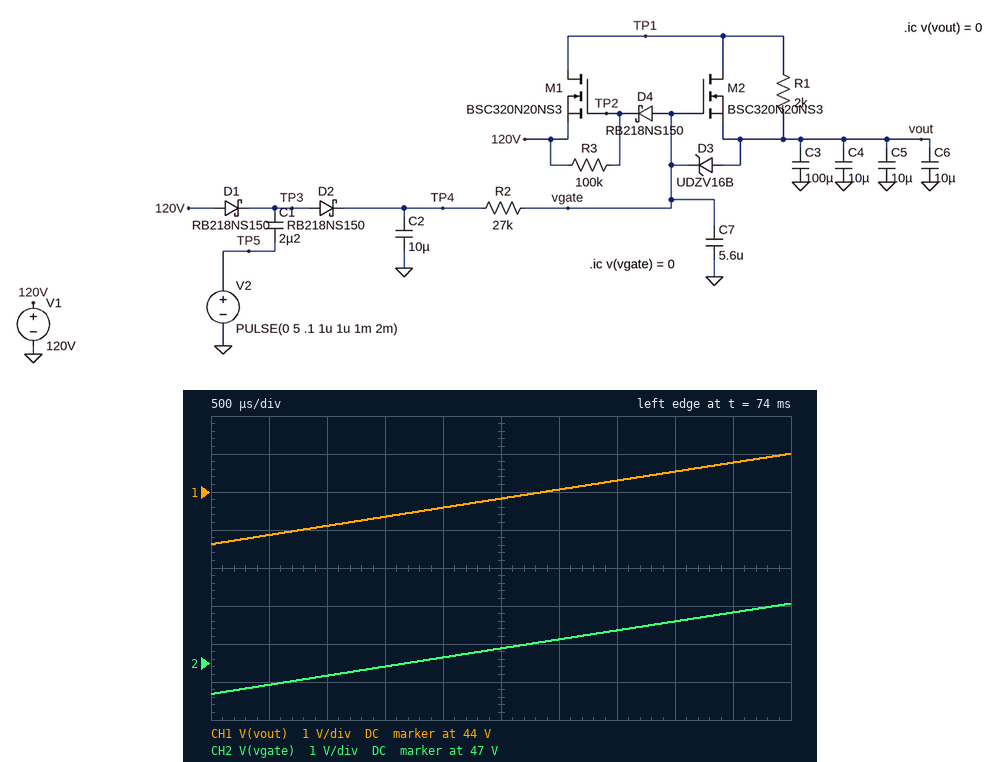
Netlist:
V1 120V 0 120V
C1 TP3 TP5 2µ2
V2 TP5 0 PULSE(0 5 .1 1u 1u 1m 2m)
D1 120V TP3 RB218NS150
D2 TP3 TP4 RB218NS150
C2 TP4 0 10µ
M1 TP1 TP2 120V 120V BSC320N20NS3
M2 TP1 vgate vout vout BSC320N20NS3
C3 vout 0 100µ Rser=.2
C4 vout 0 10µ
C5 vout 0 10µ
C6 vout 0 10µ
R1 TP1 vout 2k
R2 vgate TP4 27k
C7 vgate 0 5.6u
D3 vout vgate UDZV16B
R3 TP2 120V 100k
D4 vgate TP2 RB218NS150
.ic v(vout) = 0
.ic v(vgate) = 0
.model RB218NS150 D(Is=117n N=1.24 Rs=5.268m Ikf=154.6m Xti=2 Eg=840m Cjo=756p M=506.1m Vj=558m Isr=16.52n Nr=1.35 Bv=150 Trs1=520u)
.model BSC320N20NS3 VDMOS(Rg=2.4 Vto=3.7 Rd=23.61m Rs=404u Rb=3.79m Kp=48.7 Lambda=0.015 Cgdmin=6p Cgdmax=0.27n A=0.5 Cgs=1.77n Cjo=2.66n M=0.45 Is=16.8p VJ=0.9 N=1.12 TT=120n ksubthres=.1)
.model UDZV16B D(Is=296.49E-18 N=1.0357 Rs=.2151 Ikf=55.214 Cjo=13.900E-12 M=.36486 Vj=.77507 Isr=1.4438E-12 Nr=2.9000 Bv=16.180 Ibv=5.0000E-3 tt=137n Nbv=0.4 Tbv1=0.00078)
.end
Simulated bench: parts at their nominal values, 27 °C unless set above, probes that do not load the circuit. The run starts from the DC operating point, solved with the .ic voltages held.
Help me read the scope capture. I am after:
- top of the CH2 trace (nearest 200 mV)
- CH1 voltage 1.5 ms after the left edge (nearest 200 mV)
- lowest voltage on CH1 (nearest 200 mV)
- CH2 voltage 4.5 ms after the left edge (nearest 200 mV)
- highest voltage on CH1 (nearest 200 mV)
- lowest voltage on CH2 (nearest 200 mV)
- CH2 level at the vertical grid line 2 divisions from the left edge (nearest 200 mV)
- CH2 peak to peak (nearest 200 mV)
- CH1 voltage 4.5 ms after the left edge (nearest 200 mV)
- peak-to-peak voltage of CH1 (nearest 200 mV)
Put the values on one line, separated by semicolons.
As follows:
48.6 V; 43.4 V; 42.6 V; 48.4 V; 45.0 V; 46.2 V; 46.6 V; 2.4 V; 44.8 V; 2.4 V
